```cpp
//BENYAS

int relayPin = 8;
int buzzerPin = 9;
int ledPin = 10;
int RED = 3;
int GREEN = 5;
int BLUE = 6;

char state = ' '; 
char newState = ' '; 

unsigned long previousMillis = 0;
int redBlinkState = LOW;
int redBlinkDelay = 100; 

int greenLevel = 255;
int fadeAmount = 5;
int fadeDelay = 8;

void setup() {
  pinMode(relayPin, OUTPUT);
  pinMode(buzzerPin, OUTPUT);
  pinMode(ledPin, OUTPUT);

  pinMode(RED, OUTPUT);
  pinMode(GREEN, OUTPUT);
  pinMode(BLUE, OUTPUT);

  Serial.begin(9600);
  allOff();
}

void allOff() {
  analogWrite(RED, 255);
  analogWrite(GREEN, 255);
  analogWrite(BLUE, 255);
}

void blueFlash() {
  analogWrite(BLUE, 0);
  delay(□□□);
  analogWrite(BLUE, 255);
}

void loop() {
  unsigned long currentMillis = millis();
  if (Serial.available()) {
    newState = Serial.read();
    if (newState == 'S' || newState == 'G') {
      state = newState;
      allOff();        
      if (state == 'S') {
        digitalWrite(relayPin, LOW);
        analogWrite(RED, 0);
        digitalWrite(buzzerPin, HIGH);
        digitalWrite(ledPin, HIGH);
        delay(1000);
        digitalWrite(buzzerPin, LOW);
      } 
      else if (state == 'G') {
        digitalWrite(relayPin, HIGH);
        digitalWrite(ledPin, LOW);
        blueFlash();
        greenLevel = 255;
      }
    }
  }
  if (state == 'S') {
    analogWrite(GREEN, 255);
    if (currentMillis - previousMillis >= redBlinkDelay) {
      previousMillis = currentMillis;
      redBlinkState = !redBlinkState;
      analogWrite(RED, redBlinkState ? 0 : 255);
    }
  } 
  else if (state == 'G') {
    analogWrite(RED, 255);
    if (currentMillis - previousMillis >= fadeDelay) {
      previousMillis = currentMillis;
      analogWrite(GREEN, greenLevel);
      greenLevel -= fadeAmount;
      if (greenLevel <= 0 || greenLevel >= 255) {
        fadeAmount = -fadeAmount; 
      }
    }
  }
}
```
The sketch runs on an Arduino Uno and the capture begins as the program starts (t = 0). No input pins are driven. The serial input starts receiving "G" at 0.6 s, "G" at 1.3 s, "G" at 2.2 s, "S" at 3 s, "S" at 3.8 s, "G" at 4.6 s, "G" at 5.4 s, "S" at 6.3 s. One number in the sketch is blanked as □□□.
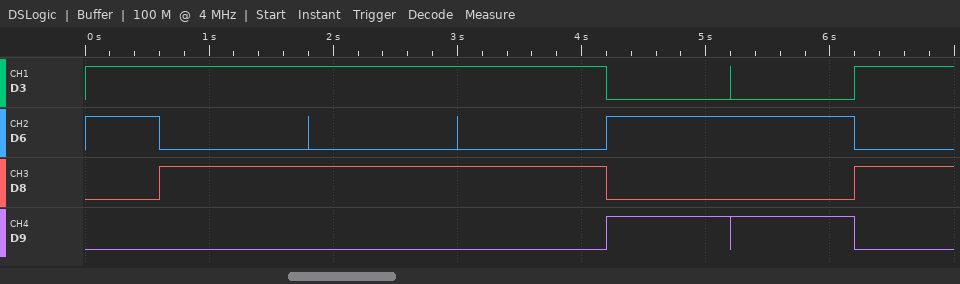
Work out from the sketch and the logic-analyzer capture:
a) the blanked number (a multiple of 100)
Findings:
1200
